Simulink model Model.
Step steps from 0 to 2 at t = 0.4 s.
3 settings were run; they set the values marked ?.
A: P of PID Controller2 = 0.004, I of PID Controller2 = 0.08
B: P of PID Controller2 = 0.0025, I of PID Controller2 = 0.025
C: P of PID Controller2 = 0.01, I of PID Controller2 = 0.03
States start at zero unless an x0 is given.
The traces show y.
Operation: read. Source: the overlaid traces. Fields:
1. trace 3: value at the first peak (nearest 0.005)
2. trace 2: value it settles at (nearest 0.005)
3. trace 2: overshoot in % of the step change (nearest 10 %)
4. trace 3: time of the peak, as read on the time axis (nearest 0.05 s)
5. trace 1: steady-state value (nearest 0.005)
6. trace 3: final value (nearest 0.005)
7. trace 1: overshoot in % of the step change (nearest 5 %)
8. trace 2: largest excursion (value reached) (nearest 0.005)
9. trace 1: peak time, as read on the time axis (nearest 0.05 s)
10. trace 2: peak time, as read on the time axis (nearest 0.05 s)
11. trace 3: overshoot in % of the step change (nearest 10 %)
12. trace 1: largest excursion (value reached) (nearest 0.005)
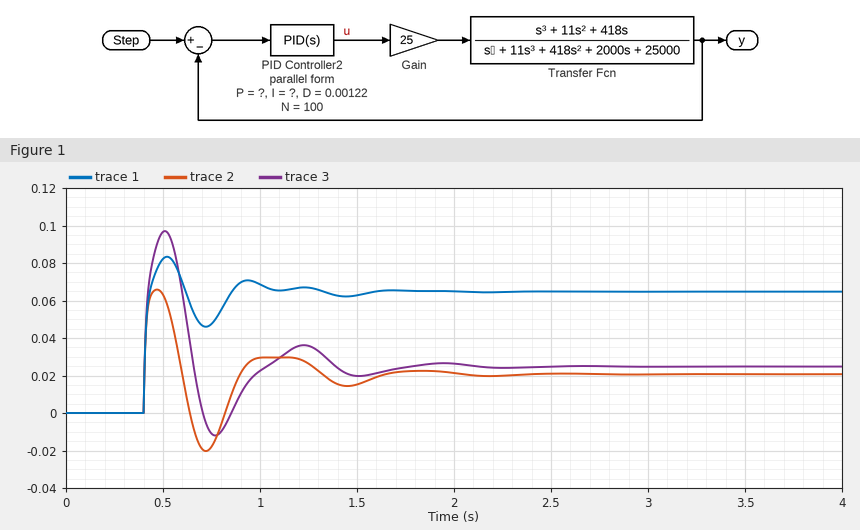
0.095
0.020
220 %
0.50 s
0.065
0.025
30 %
0.065
0.50 s
0.45 s
290 %
0.085
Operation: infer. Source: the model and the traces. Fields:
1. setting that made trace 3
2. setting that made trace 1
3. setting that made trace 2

C
A
B
